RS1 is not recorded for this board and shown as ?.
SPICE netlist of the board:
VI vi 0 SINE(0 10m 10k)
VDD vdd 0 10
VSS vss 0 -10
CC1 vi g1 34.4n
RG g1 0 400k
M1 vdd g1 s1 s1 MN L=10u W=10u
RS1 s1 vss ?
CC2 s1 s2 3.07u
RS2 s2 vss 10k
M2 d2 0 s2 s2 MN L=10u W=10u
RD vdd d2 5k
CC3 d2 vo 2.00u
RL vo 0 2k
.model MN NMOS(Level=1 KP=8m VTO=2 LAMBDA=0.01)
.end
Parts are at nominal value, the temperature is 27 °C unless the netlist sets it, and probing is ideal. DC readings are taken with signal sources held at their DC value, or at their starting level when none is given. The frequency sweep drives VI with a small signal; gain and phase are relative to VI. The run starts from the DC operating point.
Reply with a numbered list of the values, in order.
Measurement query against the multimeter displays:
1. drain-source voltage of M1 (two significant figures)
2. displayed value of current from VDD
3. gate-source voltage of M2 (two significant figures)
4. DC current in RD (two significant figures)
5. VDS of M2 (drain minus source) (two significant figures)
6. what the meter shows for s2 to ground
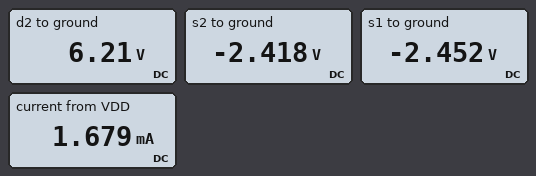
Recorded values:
1. 12 V
2. 1.679 mA
3. 2.4 V
4. 760 µA
5. 8.6 V
6. -2.418 V
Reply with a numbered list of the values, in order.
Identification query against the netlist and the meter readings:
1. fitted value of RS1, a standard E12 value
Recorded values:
1. 8.2 kΩ
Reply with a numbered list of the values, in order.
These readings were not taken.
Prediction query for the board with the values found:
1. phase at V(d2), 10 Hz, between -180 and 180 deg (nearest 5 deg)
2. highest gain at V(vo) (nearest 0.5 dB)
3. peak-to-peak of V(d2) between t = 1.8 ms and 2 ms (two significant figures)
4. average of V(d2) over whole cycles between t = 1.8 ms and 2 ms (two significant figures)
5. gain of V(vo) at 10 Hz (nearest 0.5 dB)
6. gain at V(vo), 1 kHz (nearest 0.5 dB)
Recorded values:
1. 105 deg
2. 8.5 dB
3. 53 mV
4. 6.2 V
5. -19.0 dB
6. 8.5 dB
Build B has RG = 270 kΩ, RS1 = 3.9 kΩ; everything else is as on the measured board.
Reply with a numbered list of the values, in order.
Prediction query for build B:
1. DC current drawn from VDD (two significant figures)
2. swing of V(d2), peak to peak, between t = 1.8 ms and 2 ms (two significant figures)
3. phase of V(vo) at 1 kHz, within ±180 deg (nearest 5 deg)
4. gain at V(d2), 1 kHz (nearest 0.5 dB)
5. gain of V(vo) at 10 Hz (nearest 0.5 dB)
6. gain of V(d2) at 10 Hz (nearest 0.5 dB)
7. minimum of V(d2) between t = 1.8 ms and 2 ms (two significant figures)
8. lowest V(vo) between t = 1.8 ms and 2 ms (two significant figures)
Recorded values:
1. 2.6 mA
2. 61 mV
3. 10 deg
4. 9.5 dB
5. -21.5 dB
6. -9.0 dB
7. 6.2 V
8. -31 mV
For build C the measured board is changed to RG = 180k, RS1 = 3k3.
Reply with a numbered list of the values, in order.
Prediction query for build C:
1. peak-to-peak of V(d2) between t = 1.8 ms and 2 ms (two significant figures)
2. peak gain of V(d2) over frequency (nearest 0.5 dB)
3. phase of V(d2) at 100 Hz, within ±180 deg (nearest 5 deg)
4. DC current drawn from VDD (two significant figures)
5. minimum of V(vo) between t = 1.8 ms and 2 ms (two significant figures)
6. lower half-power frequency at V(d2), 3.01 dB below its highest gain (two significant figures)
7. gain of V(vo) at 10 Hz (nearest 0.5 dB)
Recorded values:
1. 63 mV
2. 10.0 dB
3. 50 deg
4. 3.0 mA
5. -32 mV
6. 120 Hz
7. -24.5 dB
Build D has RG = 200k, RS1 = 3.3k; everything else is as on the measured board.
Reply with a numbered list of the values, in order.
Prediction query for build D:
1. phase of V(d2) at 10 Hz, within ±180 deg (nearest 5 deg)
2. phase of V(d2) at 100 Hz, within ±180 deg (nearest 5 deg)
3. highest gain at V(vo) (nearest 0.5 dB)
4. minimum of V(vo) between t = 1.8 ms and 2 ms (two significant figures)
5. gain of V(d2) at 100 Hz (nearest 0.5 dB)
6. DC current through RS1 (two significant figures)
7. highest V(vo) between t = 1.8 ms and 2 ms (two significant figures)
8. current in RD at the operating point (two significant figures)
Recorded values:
1. 125 deg
2. 50 deg
3. 10.0 dB
4. -32 mV
5. 6.5 dB
6. 2.2 mA
7. 31 mV
8. 760 µA
